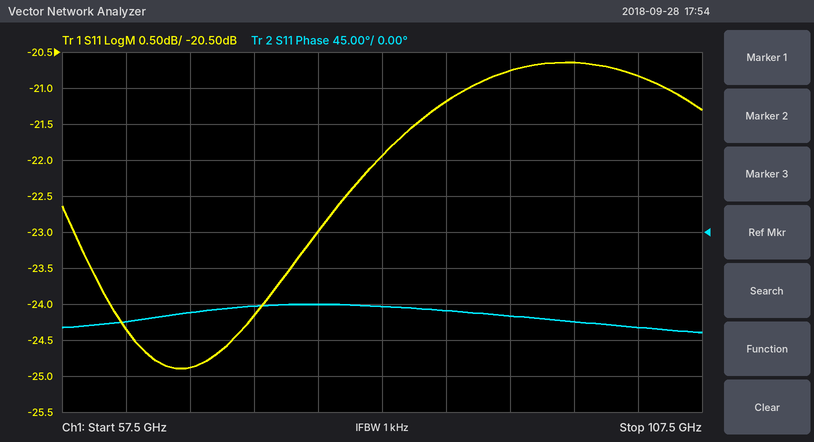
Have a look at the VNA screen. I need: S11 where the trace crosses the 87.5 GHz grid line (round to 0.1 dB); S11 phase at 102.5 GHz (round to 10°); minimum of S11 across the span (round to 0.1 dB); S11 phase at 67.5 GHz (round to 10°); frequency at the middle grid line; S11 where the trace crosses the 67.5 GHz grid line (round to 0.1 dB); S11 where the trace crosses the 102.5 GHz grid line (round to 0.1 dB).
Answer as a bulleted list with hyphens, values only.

- -21.2 dB
- -120°
- -24.9 dB
- -100°
- 82.5 GHz
- -24.9 dB
- -20.8 dB
